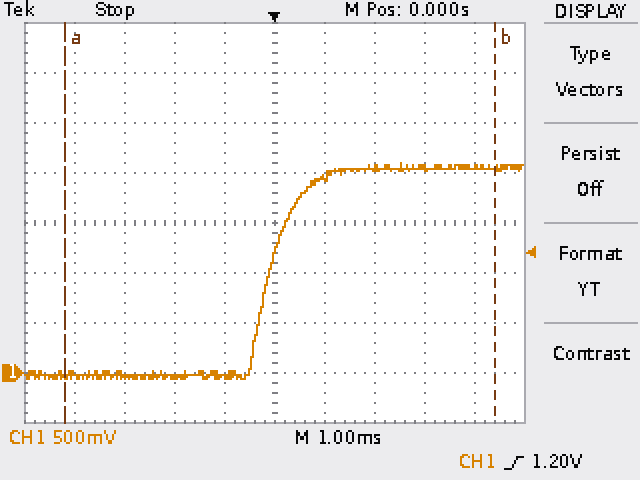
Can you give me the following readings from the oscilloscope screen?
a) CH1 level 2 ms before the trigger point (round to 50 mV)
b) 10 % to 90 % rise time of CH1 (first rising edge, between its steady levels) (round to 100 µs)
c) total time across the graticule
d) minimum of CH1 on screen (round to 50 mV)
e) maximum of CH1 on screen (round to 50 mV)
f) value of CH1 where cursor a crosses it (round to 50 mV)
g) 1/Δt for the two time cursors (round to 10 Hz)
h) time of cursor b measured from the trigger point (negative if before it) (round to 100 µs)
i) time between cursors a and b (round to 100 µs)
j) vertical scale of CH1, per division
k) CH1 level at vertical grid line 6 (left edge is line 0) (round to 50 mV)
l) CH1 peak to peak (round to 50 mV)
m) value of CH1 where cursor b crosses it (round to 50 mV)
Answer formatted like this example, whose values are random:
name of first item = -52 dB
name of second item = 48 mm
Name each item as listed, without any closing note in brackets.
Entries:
CH1 level 2 ms before the trigger point = -50 mV
10 % to 90 % rise time of CH1 (first rising edge, between its steady levels) = 1.1 ms
total time across the graticule = 10 ms
minimum of CH1 on screen = -50 mV
maximum of CH1 on screen = 2.10 V
value of CH1 where cursor a crosses it = 0 mV
1/Δt for the two time cursors = 120 Hz
time of cursor b measured from the trigger point (negative if before it) = +4.4 ms
time between cursors a and b = 8.6 ms
vertical scale of CH1, per division = 500 mV
CH1 level at vertical grid line 6 (left edge is line 0) = 1.95 V
CH1 peak to peak = 2.15 V
value of CH1 where cursor b crosses it = 2.05 V
